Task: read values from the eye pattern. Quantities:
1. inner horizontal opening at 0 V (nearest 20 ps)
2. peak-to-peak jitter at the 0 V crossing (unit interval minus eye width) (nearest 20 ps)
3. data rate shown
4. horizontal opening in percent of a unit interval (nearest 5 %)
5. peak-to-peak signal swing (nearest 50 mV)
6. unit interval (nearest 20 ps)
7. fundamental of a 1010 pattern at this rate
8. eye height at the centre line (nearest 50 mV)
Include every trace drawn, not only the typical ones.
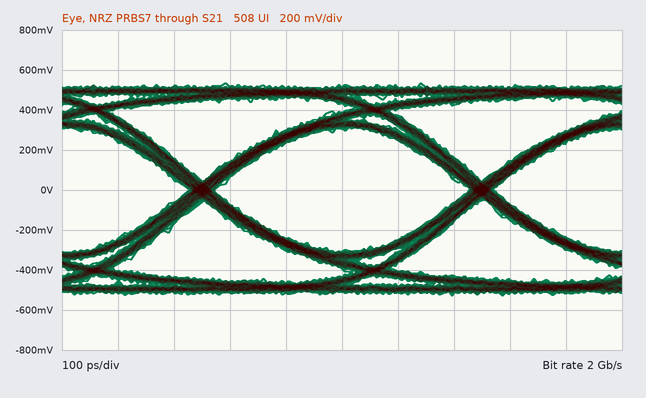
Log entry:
460 ps
40 ps
2 Gb/s
90 %
1.05 V
500 ps
1 GHz
600 mV
